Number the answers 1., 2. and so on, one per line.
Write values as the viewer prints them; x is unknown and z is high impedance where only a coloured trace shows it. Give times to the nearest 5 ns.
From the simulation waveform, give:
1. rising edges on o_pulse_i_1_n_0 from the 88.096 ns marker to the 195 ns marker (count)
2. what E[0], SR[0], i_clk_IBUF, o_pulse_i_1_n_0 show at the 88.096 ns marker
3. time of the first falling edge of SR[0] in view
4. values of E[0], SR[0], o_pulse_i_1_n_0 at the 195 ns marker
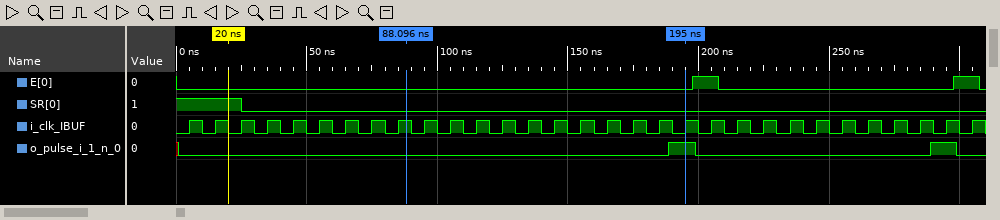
1. 1
2. E[0]=0, SR[0]=0, i_clk_IBUF=1, o_pulse_i_1_n_0=0
3. 25 ns
4. E[0]=0, SR[0]=0, o_pulse_i_1_n_0=1
